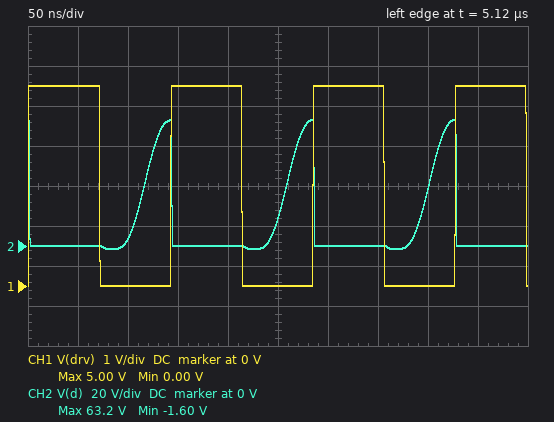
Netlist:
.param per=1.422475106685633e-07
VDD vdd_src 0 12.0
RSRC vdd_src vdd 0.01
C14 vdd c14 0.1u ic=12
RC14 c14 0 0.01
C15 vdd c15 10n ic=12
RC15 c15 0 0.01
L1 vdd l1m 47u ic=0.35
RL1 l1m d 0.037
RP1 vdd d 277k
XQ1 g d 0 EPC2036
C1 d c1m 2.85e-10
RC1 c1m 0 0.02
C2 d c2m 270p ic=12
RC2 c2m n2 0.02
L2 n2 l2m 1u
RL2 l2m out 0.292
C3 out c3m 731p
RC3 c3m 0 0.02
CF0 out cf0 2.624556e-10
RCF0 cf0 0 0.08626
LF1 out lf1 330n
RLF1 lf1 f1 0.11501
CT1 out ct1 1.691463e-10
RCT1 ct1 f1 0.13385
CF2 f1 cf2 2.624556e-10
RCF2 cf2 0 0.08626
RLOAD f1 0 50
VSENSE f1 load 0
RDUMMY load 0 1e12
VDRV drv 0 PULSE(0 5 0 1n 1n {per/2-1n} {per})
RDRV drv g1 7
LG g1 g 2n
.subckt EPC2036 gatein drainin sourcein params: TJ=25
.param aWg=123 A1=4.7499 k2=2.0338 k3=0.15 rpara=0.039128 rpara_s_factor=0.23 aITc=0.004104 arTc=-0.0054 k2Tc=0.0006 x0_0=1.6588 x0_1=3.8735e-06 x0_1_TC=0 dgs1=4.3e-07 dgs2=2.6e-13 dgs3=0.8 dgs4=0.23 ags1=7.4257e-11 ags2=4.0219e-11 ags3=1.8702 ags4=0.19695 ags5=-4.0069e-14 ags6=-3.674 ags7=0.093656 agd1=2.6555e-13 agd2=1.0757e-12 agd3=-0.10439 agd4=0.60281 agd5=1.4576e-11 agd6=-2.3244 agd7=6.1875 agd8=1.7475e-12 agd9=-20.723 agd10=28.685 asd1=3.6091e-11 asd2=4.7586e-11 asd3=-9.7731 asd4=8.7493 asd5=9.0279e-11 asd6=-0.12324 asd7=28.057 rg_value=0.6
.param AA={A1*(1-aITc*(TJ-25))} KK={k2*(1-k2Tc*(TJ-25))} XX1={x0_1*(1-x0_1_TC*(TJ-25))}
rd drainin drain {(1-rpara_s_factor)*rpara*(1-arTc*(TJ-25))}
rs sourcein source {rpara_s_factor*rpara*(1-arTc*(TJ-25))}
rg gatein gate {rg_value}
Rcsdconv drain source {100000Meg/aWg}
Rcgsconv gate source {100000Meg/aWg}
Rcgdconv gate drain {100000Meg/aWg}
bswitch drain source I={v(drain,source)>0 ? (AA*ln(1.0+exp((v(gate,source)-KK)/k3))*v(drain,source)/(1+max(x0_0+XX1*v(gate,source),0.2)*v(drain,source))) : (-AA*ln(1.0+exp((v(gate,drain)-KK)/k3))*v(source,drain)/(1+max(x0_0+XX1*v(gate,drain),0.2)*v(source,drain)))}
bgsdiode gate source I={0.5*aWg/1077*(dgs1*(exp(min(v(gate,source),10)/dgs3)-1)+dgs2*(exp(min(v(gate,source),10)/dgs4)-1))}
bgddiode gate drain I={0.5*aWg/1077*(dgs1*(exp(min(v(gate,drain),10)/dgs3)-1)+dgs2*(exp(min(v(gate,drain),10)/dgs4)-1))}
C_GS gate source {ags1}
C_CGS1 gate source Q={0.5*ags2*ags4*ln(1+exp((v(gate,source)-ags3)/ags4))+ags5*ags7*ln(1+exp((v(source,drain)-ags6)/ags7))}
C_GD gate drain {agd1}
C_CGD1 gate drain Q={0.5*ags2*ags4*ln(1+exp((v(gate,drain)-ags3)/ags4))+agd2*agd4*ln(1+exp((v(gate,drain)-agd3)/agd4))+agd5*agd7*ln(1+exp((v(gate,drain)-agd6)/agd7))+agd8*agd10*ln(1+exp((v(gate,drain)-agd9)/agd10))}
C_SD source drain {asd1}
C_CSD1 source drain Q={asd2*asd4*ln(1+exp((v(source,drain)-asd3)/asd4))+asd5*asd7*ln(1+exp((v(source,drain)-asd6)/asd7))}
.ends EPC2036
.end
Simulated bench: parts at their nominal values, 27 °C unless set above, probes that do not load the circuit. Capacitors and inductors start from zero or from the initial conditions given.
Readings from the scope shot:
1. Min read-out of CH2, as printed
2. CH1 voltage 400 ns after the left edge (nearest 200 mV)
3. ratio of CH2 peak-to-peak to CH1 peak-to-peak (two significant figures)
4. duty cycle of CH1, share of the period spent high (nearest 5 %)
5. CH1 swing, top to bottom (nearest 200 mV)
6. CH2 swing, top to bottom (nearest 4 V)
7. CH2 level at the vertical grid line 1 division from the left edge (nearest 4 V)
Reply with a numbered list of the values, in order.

1. -1.60 V
2. 0 V
3. 13
4. 50 %
5. 5.0 V
6. 64 V
7. 0 V
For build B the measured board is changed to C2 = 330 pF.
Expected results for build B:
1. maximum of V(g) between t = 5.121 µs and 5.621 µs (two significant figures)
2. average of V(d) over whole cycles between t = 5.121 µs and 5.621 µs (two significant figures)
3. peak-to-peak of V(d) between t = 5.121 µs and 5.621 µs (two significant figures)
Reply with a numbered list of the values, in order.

1. 5.0 V
2. 11 V
3. 68 V
